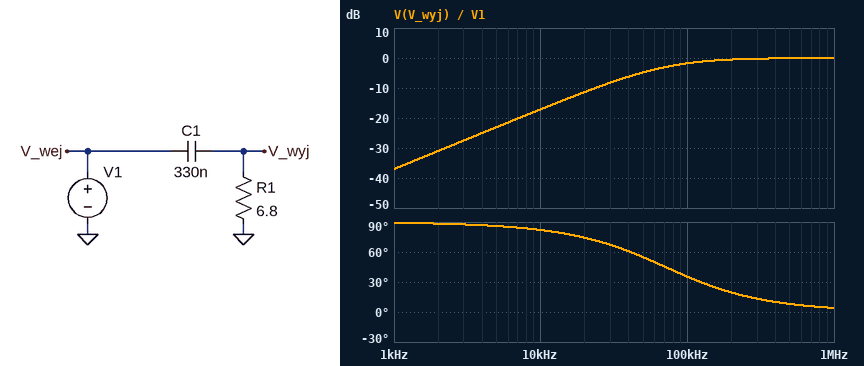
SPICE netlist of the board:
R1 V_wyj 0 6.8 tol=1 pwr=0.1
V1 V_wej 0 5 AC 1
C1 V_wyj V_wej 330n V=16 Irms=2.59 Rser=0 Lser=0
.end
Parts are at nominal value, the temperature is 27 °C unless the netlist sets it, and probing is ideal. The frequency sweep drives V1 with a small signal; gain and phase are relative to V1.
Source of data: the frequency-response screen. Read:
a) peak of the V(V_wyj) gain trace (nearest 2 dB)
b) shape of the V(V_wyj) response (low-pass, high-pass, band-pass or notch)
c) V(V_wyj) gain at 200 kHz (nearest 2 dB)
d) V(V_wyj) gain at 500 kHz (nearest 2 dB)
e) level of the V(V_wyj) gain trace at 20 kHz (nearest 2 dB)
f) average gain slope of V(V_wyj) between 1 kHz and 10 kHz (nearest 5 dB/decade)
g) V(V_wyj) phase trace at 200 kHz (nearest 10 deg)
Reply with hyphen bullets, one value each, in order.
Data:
- 0 dB
- high-pass
- 0 dB
- 0 dB
- -12 dB
- 20 dB/decade
- 20 deg
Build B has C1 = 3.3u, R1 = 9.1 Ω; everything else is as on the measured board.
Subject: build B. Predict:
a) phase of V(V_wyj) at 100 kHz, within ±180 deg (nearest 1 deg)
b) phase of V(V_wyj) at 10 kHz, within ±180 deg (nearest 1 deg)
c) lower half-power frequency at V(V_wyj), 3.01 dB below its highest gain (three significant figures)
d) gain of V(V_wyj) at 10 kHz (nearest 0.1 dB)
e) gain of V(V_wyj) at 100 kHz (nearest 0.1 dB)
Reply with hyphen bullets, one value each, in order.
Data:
- 3 deg
- 28 deg
- 5.30 kHz
- -1.1 dB
- 0 dB
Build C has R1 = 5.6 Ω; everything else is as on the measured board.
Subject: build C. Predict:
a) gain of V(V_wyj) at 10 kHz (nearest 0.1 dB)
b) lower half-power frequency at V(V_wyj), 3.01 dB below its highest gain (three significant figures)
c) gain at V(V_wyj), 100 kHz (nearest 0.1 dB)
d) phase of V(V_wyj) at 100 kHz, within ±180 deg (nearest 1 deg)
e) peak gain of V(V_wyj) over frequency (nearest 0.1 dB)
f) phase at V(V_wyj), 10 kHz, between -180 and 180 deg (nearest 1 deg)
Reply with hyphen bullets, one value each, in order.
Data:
- -18.8 dB
- 86.1 kHz
- -2.4 dB
- 41 deg
- 0 dB
- 83 deg
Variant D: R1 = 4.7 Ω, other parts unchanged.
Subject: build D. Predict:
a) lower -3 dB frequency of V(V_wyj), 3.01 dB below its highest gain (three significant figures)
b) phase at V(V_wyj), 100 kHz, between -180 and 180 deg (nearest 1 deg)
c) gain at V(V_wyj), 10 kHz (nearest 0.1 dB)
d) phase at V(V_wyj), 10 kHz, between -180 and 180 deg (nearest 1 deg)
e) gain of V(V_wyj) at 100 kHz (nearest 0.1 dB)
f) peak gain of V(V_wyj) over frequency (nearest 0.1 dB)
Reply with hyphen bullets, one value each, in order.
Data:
- 103 kHz
- 46 deg
- -20.3 dB
- 84 deg
- -3.1 dB
- 0 dB
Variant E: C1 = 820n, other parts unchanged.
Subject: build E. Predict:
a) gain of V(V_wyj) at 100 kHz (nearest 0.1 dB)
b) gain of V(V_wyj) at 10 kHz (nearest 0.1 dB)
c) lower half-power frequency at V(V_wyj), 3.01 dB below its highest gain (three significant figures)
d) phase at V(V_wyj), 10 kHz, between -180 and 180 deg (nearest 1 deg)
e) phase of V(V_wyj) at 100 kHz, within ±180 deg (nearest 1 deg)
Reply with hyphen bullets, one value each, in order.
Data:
- -0.3 dB
- -9.6 dB
- 28.5 kHz
- 71 deg
- 16 deg
